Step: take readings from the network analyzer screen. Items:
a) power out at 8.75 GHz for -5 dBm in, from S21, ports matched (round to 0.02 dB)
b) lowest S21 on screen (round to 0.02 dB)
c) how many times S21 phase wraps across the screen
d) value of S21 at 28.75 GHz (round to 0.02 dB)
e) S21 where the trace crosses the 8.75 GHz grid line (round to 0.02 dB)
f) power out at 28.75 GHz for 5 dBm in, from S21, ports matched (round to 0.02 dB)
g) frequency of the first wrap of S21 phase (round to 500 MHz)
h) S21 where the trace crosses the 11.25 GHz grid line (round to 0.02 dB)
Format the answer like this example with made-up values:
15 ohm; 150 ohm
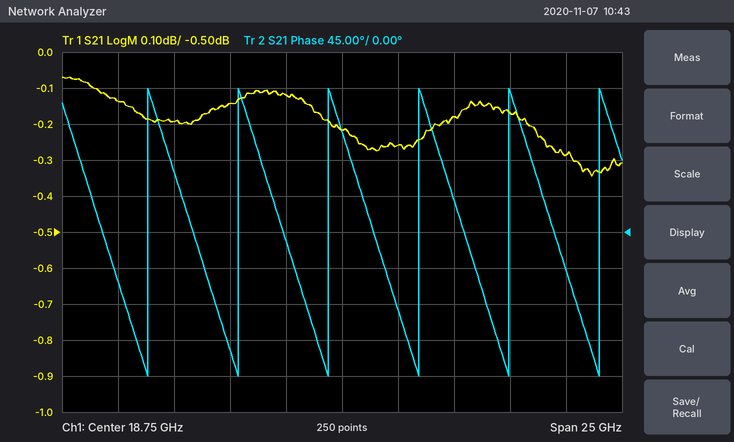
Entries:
-5.14 dBm; -0.34 dB; 6; -0.28 dB; -0.14 dB; 4.72 dBm; 10.0 GHz; -0.20 dB
